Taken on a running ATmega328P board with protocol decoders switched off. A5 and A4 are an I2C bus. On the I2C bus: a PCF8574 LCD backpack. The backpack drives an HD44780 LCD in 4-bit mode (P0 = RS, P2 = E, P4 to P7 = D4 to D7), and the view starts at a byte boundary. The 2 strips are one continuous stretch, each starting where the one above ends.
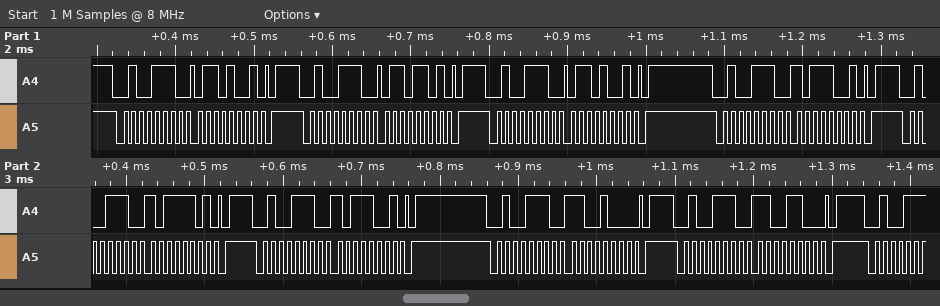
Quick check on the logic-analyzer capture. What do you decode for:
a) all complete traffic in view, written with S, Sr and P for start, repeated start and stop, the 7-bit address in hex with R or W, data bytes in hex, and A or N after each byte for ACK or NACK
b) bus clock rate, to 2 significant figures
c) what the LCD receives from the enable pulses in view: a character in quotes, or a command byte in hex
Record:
S 27W A 69 A P S 27W A 6D A P S 27W A 69 A P S 27W A B9 A P S 27W A BD A P S 27W A B9 A P S 27W A C8 A P S 27W A CC A P
100 kHz
'k'
